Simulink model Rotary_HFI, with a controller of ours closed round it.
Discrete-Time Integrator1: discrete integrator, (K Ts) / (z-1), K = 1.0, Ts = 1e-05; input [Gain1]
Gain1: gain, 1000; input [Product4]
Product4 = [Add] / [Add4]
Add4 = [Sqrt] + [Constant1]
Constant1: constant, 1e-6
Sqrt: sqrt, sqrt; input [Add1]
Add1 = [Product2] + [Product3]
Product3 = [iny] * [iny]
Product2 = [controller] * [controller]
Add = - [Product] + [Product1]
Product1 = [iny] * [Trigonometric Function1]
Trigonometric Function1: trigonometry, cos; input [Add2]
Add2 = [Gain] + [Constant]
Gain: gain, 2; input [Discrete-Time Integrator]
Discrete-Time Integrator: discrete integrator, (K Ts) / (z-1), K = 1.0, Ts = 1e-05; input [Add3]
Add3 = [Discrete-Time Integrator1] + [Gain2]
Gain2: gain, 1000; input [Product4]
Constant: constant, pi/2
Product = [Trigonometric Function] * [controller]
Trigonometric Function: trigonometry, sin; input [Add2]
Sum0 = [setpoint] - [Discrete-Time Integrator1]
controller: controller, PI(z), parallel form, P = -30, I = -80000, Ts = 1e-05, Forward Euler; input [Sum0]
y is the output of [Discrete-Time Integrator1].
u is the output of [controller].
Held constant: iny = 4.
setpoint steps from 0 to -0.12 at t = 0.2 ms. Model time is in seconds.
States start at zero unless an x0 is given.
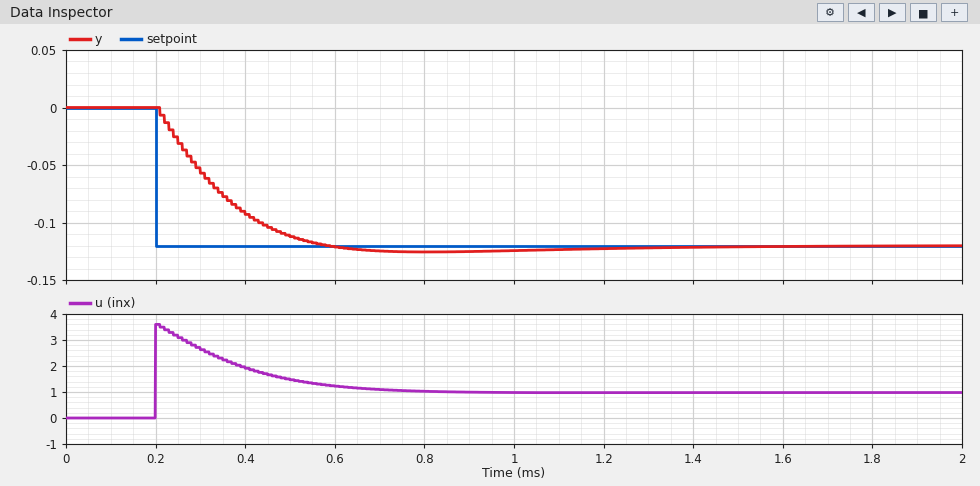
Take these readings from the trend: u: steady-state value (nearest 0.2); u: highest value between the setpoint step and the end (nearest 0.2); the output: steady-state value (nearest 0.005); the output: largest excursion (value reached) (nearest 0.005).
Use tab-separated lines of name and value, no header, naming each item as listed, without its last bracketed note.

u: steady-state value	1.0
u: highest value between the setpoint step and the end	3.6
the output: steady-state value	-0.120
the output: largest excursion (value reached)	-0.125
